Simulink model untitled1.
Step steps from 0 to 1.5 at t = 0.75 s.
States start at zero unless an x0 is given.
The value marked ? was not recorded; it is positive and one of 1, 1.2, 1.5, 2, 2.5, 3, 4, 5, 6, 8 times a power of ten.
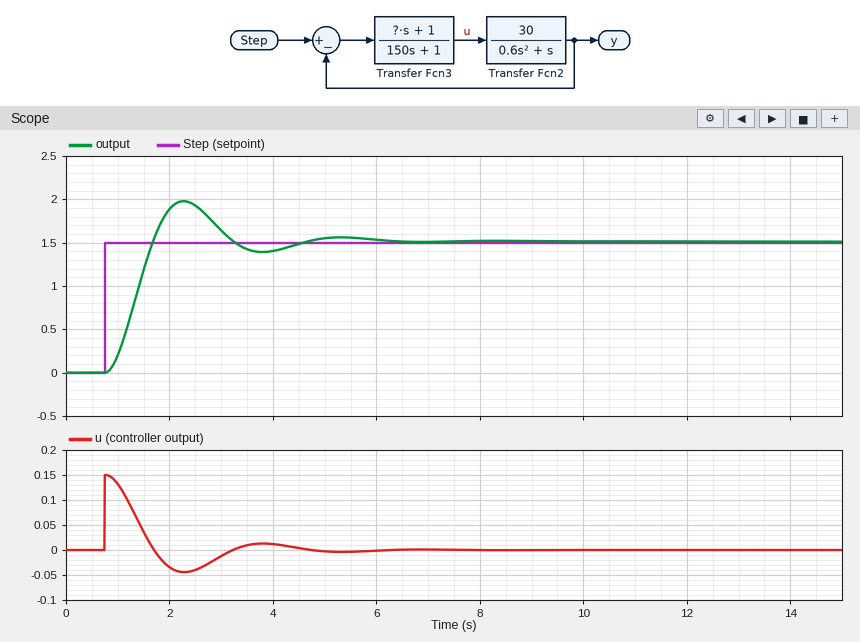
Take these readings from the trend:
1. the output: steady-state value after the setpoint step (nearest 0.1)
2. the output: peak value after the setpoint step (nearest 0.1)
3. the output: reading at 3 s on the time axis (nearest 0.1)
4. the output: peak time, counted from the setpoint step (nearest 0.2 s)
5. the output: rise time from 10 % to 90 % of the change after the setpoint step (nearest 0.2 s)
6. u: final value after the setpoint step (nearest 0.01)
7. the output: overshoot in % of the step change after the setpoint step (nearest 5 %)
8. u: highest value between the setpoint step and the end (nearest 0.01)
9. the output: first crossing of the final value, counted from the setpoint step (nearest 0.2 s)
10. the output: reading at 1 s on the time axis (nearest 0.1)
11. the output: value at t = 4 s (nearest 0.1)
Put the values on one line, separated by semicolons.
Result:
1.5; 2.0; 1.6; 1.6 s; 0.6 s; 0.00; 30 %; 0.15; 1.0 s; 0.2; 1.4
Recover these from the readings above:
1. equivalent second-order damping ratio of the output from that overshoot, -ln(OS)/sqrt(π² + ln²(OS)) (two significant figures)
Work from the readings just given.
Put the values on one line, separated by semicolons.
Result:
0.36
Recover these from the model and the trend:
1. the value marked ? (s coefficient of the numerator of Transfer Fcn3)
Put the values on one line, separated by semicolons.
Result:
15
